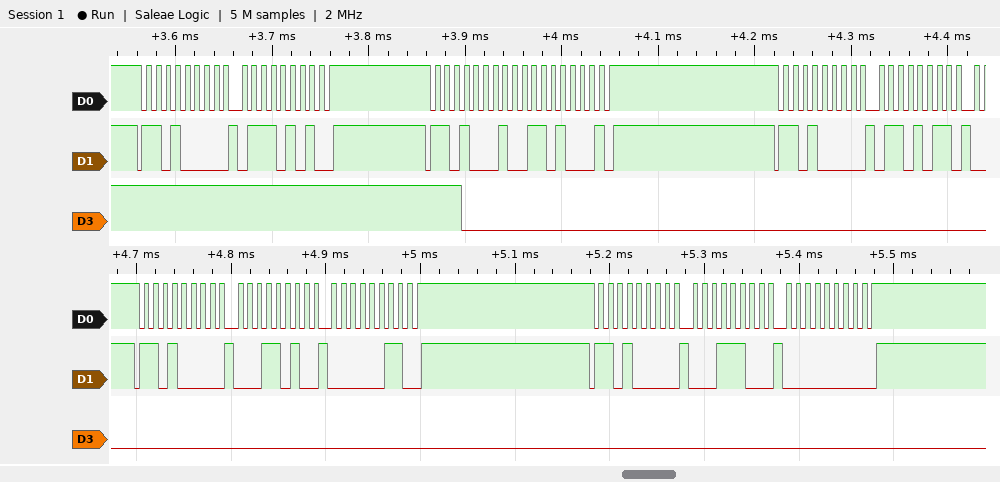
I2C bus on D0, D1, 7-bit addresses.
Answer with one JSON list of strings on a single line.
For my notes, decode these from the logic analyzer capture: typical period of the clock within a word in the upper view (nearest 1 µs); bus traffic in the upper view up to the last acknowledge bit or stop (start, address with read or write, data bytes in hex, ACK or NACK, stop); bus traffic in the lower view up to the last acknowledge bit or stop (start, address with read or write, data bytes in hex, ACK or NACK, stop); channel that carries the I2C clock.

["10 µs", "start, address 68 write ACK, 75 ACK, stop, start, address 68 read ACK, 68 NACK, stop, start, address 68 write ACK, 6B ACK", "start, address 68 write ACK, 1A ACK, 03 ACK, stop, start, address 68 write ACK, 1C ACK, 00 ACK, stop", "D0"]
